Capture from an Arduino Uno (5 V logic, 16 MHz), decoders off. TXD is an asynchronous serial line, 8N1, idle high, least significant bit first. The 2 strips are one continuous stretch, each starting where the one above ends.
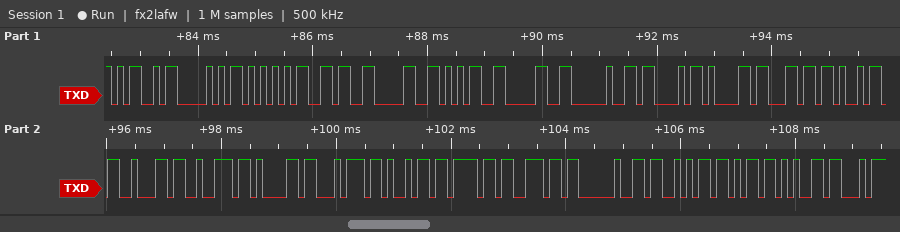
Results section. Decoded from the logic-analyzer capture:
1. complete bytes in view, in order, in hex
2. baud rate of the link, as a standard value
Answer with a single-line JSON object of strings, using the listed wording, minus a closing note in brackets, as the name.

{"complete bytes in view, in order, in hex": "4D 50 55 36 30 35 30 20 43 61 6C 69 62 72 61 74 69 6F 6E 20 53 6B 65", "baud rate of the link, as a standard value": "9600 baud"}
